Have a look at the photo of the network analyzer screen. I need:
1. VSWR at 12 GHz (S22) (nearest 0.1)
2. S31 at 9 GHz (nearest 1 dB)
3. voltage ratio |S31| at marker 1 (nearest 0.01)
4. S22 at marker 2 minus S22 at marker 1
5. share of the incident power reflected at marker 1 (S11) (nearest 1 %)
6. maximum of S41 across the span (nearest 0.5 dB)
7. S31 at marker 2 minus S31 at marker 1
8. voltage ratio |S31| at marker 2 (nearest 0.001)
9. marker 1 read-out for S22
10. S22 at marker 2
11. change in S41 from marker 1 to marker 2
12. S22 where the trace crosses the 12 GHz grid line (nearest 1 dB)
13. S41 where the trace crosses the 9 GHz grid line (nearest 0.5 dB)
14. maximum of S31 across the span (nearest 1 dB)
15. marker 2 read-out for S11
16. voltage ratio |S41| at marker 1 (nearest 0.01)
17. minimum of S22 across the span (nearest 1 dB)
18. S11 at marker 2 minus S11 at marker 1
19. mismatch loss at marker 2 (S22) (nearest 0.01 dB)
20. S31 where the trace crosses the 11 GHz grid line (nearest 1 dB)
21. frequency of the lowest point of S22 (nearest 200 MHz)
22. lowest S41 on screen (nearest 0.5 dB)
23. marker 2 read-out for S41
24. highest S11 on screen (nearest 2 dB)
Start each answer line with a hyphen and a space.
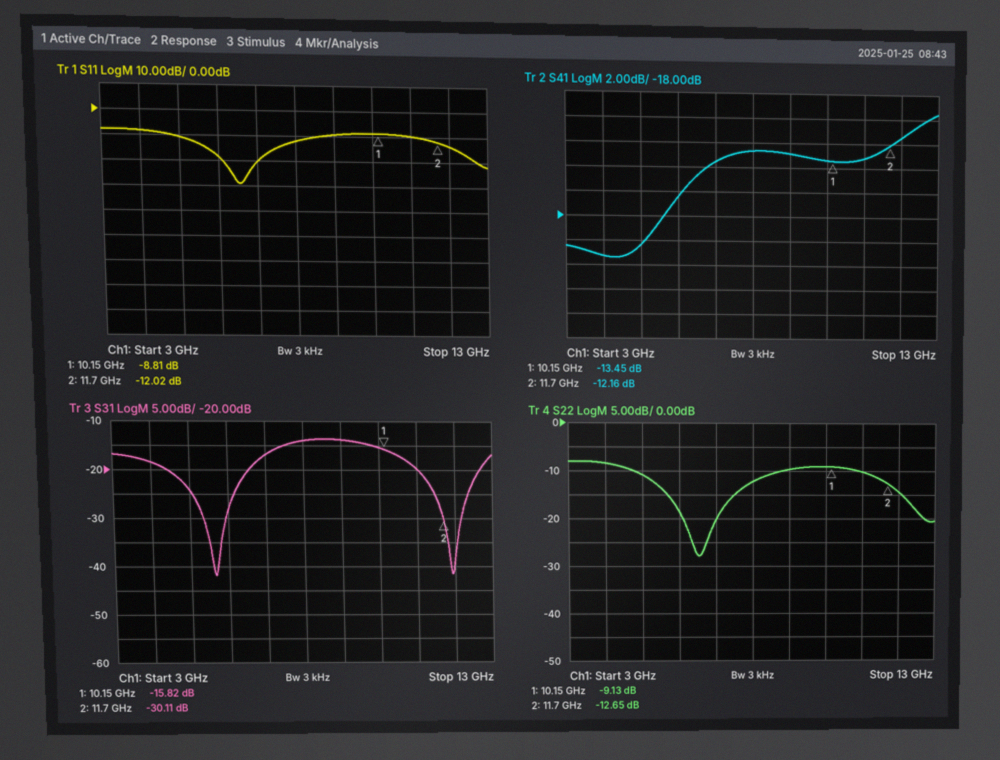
- 1.5
- -14 dB
- 0.16
- -3.52 dB
- 13 %
- -9.5 dB
- -14.29 dB
- 0.031
- -9.13 dB
- -12.65 dB
- 1.29 dB
- -14 dB
- -13.0 dB
- -14 dB
- -12.02 dB
- 0.21
- -28 dB
- -3.21 dB
- 0.24 dB
- -20 dB
- 6.6 GHz
- -21.5 dB
- -12.16 dB
- -8 dB
